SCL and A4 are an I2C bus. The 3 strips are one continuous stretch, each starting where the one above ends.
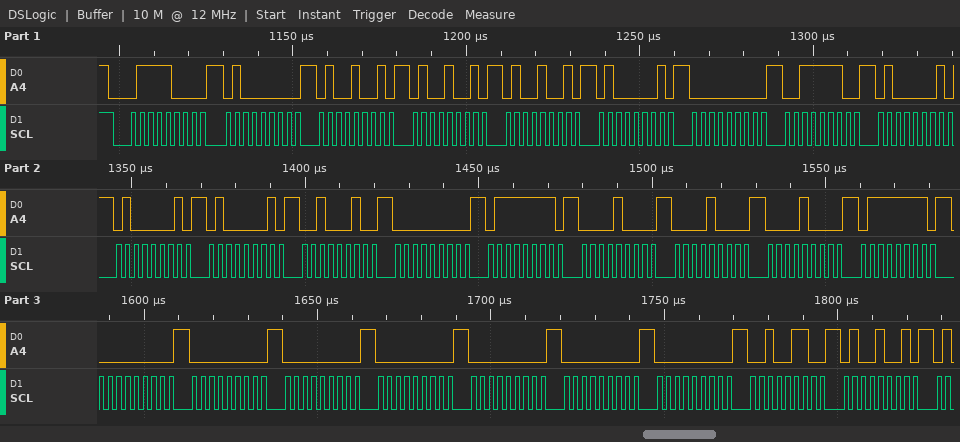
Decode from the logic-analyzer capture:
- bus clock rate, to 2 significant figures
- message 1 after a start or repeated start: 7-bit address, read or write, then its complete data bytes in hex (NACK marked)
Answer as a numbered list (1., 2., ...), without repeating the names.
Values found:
1. 400 kHz
2. 0x3C write: 40 49 49 49 41 00 3E 41 41 41 22 00 7F 08 08 08 7F 00 00 00 00 00 00 00 26 49
